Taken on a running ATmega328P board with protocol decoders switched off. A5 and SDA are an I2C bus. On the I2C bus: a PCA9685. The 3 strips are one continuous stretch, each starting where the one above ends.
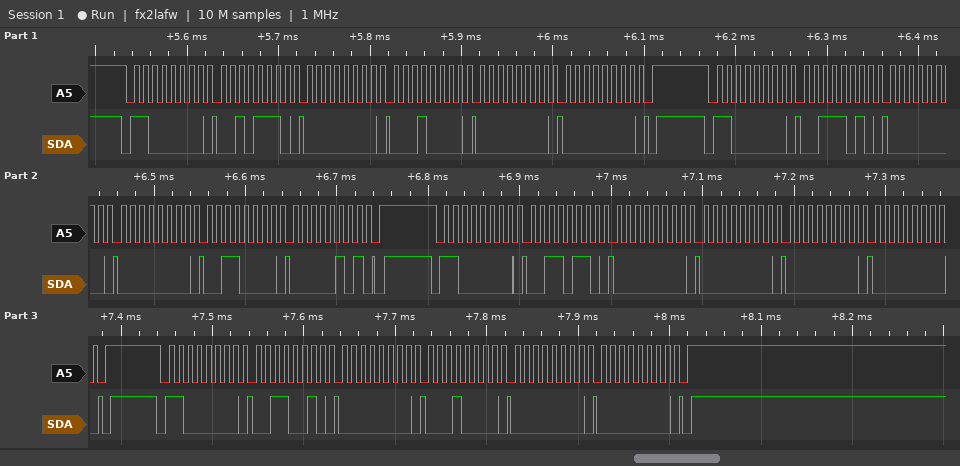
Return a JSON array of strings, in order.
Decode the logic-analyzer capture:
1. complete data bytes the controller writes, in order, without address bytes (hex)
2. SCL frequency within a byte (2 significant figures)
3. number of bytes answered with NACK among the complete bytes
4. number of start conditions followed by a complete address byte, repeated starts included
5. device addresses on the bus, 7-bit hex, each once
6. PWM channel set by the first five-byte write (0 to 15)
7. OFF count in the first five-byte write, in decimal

["2E 00 10 00 00 3A 00 00 30 05 36 00 00 00 00 32 00 10 00 00", "100 kHz", "0", "4", "0x60", "10", "0"]
